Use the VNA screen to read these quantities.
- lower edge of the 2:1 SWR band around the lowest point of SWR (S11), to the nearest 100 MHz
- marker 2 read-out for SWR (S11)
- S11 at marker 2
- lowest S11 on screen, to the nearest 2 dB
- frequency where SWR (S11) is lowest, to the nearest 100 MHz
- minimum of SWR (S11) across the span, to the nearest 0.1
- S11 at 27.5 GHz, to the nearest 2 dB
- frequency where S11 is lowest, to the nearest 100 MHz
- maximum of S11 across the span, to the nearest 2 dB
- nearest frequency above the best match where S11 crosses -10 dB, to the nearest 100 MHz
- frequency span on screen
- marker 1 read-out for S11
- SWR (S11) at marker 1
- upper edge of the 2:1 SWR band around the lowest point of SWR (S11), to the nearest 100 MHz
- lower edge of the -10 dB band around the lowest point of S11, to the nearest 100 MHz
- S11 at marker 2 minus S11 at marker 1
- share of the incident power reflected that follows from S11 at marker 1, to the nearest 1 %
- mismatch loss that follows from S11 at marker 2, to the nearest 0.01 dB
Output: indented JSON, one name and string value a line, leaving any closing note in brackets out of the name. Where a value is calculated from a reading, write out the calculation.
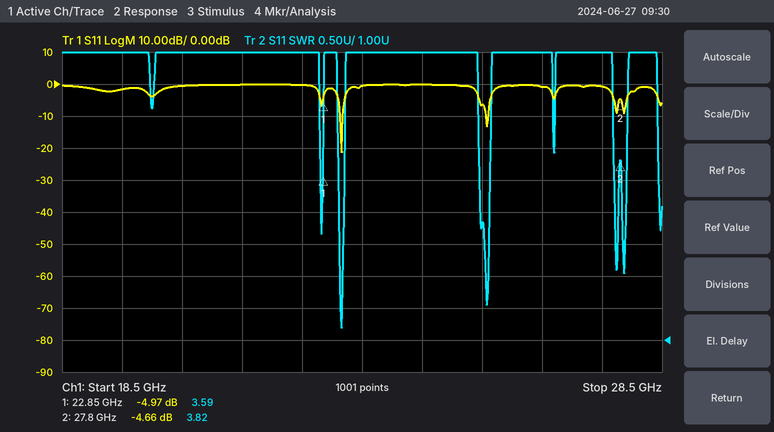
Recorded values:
{
  "lower edge of the 2:1 SWR band around the lowest point of SWR (S11), to the nearest 100 MHz": "23.1 GHz",
  "marker 2 read-out for SWR": "3.82",
  "S11 at marker 2": "-4.66 dB",
  "lowest S11 on screen, to the nearest 2 dB": "-22 dB",
  "frequency where SWR (S11) is lowest, to the nearest 100 MHz": "23.2 GHz",
  "minimum of SWR (S11) across the span, to the nearest 0.1": "1.2",
  "S11 at 27.5 GHz, to the nearest 2 dB": "0 dB",
  "frequency where S11 is lowest, to the nearest 100 MHz": "23.2 GHz",
  "maximum of S11 across the span, to the nearest 2 dB": "0 dB",
  "nearest frequency above the best match where S11 crosses -10 dB, to the nearest 100 MHz": "23.2 GHz",
  "frequency span on screen": "10 GHz",
  "marker 1 read-out for S11": "-4.97 dB",
  "SWR (S11) at marker 1": "3.59",
  "upper edge of the 2:1 SWR band around the lowest point of SWR (S11), to the nearest 100 MHz": "23.2 GHz",
  "lower edge of the -10 dB band around the lowest point of S11, to the nearest 100 MHz": "23.1 GHz",
  "S11 at marker 2 minus S11 at marker 1": "-4.66 − (-4.97) = 0.31 dB",
  "share of the incident power reflected that follows from S11 at marker 1, to the nearest 1 %": "10^(-4.97/10) ≈ 32 %",
  "mismatch loss that follows from S11 at marker 2, to the nearest 0.01 dB": "−10 log10(1 − 10^(-4.66/10)) ≈ 1.82 dB"
}
